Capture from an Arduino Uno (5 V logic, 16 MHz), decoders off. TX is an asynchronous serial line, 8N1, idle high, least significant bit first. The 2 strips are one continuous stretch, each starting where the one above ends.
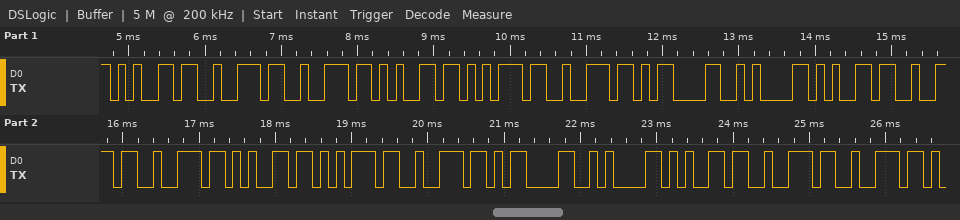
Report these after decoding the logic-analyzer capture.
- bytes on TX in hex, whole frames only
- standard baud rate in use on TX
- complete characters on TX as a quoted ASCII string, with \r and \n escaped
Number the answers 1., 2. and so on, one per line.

1. 65 72 72 65 75 72 0D 0A 65 72 72 65 75 72 0D 0A 65 72 72
2. 9600 baud
3. "erreur\r\nerreur\r\nerr"
